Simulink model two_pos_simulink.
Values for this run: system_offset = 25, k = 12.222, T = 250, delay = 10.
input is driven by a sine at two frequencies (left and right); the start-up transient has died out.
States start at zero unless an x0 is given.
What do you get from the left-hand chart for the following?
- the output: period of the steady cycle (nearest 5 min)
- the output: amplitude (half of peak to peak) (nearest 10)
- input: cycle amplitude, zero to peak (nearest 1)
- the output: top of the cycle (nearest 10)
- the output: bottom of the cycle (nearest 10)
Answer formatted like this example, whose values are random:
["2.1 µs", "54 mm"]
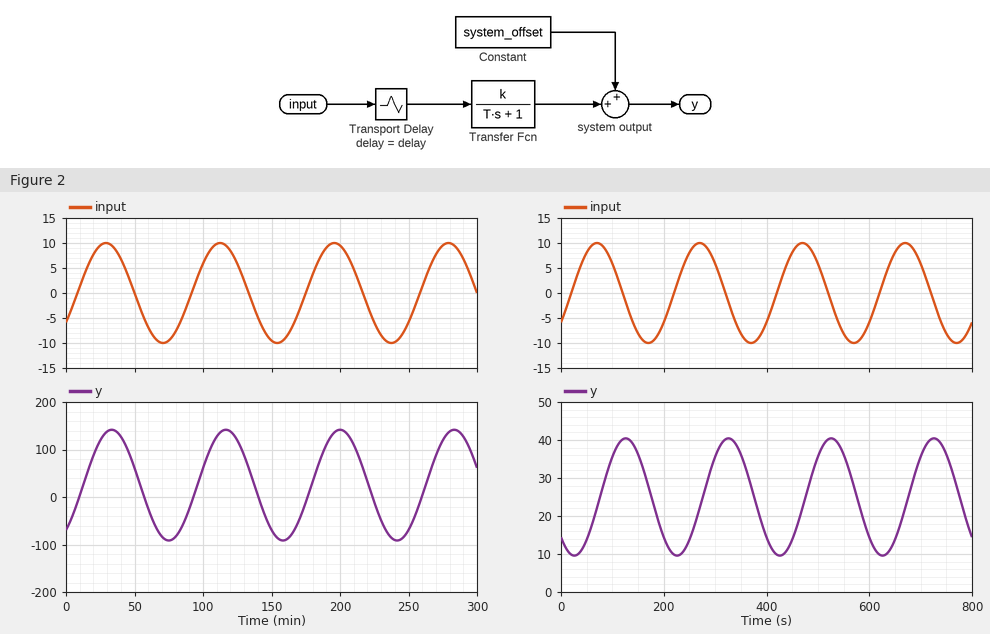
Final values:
["85 min", "120", "10", "140", "-90"]
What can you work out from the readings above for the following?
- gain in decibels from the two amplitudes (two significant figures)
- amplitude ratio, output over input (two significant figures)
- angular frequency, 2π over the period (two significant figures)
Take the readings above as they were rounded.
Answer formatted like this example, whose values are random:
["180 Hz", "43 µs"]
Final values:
["22 dB", "12", "0.074 rad/min"]
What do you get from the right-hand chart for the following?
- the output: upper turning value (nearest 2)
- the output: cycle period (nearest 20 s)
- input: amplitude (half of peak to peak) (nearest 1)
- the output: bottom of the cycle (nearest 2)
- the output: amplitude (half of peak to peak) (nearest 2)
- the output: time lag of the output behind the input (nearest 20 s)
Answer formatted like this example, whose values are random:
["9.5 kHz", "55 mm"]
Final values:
["40", "200 s", "10", "10", "16", "60 s"]
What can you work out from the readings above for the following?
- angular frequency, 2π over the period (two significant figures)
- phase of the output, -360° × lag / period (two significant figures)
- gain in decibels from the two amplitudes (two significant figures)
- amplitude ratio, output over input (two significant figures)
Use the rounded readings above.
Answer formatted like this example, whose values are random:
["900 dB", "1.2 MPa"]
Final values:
["0.031 rad/s", "-110°", "4.1 dB", "1.6"]
